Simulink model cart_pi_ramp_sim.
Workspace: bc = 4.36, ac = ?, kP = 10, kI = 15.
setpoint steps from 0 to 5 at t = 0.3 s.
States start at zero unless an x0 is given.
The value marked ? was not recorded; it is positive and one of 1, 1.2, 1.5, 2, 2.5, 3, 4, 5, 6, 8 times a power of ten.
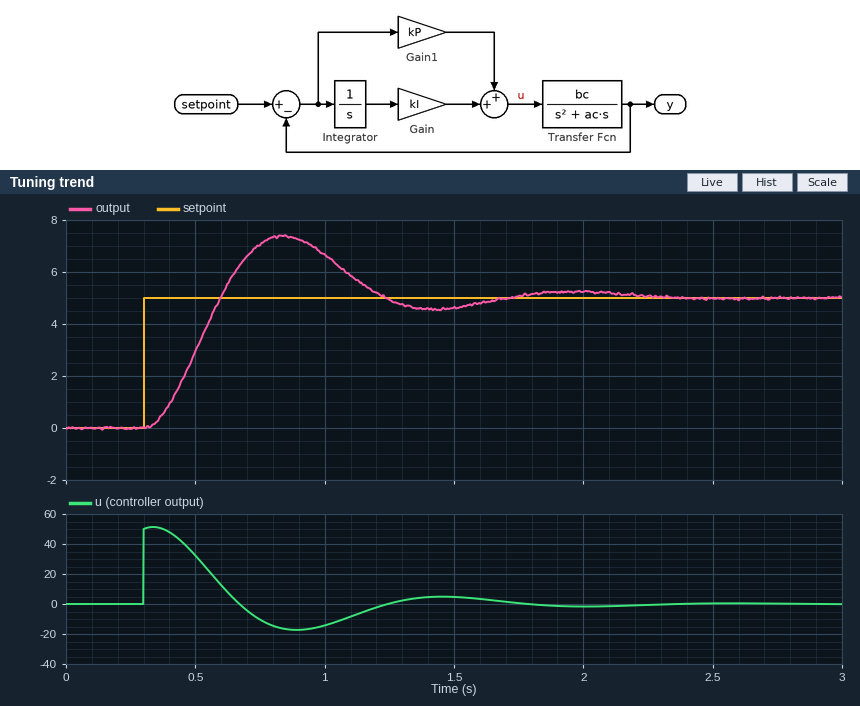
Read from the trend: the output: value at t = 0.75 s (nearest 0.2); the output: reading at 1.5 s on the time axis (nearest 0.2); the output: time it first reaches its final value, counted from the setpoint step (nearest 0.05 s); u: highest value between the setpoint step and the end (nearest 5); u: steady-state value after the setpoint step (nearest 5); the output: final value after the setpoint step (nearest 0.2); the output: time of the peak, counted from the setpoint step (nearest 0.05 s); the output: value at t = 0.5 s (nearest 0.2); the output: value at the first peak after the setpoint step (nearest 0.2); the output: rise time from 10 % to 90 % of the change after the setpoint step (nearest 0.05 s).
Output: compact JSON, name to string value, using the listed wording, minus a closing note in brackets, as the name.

{"the output: value at t = 0.75 s": "7.0", "the output: reading at 1.5 s on the time axis": "4.6", "the output: time it first reaches its final value, counted from the setpoint step": "0.30 s", "u: highest value between the setpoint step and the end": "50", "u: steady-state value after the setpoint step": "0", "the output: final value after the setpoint step": "5.0", "the output: time of the peak, counted from the setpoint step": "0.55 s", "the output: value at t = 0.5 s": "3.0", "the output: value at the first peak after the setpoint step": "7.4", "the output: rise time from 10 % to 90 % of the change after the setpoint step": "0.20 s"}
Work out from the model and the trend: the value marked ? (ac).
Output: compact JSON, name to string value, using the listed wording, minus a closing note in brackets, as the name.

{"the value marked ?": "6"}
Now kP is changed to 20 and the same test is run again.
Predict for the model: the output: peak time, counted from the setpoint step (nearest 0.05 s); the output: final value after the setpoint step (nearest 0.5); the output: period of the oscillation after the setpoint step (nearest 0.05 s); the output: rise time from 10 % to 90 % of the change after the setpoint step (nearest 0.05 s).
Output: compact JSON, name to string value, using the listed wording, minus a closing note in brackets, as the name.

{"the output: peak time, counted from the setpoint step": "0.35 s", "the output: final value after the setpoint step": "5.0", "the output: period of the oscillation after the setpoint step": "0.70 s", "the output: rise time from 10 % to 90 % of the change after the setpoint step": "0.15 s"}
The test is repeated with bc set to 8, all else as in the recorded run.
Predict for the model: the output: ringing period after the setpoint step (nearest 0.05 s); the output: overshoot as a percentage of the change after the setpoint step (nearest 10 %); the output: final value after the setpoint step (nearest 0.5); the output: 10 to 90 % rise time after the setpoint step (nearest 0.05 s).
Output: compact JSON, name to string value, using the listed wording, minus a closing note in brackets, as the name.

{"the output: ringing period after the setpoint step": "0.75 s", "the output: overshoot as a percentage of the change after the setpoint step": "50 %", "the output: final value after the setpoint step": "5.0", "the output: 10 to 90 % rise time after the setpoint step": "0.15 s"}
